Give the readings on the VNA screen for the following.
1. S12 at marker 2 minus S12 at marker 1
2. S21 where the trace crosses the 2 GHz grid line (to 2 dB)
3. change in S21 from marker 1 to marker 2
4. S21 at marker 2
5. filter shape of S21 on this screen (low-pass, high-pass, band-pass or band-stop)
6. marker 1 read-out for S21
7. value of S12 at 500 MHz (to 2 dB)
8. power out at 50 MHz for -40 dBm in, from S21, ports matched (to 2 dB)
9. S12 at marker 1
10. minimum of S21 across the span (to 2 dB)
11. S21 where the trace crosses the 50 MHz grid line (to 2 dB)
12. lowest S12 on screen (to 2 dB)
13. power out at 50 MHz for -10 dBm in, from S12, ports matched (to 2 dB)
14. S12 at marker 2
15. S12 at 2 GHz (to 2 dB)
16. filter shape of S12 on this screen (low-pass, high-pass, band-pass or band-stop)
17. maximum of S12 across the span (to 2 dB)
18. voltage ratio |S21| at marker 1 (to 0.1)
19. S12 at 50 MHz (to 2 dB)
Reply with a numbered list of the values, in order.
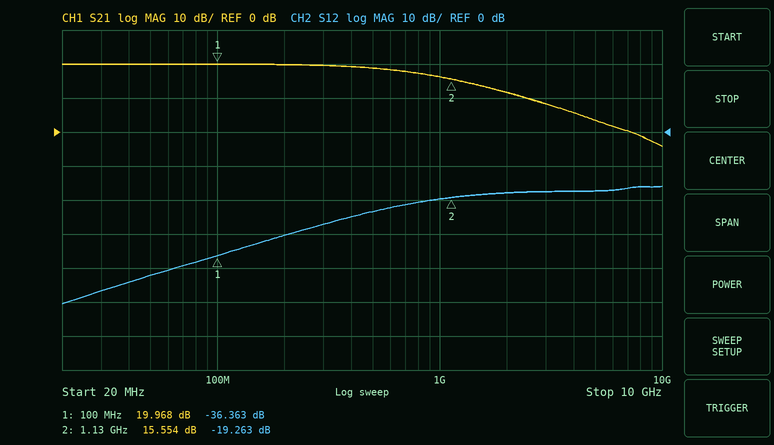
1. 17.100 dB
2. 12 dB
3. -4.414 dB
4. 15.554 dB
5. low-pass
6. 19.968 dB
7. -24 dB
8. -20 dBm
9. -36.363 dB
10. -4 dB
11. 20 dB
12. -50 dB
13. -52 dBm
14. -19.263 dB
15. -18 dB
16. high-pass
17. -16 dB
18. 10.0
19. -42 dB
